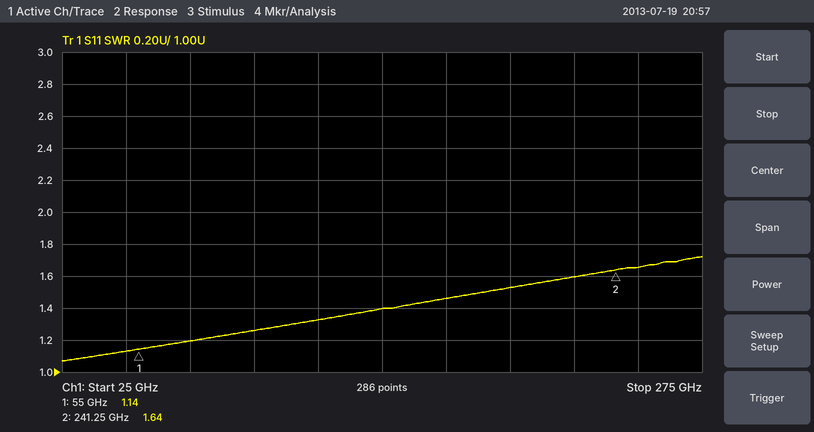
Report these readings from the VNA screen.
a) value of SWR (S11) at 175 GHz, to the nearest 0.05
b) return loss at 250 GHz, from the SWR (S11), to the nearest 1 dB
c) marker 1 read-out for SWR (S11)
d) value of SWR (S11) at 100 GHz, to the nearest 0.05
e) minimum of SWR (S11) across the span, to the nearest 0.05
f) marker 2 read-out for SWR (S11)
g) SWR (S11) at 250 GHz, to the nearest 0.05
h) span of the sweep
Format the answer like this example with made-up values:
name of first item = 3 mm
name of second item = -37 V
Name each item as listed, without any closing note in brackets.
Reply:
value of SWR (S11) at 175 GHz, to the nearest 0.05 = 1.45
return loss at 250 GHz, from the SWR (S11), to the nearest 1 dB = 12 dB
marker 1 read-out for SWR = 1.14
value of SWR (S11) at 100 GHz, to the nearest 0.05 = 1.25
minimum of SWR (S11) across the span, to the nearest 0.05 = 1.05
marker 2 read-out for SWR = 1.64
SWR (S11) at 250 GHz, to the nearest 0.05 = 1.65
span of the sweep = 250 GHz
